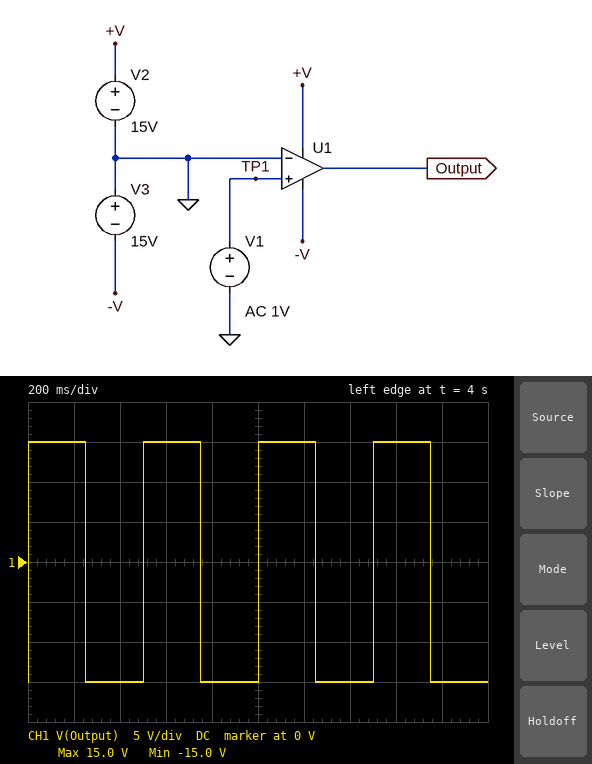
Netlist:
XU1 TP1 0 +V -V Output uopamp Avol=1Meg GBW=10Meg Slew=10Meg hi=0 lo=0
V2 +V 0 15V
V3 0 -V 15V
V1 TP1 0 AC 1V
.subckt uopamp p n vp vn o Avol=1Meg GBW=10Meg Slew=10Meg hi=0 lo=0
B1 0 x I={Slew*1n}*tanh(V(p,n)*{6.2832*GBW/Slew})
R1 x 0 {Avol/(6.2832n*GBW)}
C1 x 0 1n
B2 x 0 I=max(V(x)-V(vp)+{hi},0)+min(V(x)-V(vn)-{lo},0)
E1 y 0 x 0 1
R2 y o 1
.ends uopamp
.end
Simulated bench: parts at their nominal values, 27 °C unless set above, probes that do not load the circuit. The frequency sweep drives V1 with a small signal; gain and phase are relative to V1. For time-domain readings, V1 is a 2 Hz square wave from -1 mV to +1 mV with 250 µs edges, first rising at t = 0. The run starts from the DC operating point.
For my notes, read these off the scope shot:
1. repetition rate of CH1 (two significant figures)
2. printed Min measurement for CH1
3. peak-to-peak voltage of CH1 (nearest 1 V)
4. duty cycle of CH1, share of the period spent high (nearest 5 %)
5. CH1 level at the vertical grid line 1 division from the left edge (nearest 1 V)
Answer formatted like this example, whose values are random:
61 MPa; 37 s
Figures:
2.0 Hz; -15.0 V; 30 V; 50 %; 15 V
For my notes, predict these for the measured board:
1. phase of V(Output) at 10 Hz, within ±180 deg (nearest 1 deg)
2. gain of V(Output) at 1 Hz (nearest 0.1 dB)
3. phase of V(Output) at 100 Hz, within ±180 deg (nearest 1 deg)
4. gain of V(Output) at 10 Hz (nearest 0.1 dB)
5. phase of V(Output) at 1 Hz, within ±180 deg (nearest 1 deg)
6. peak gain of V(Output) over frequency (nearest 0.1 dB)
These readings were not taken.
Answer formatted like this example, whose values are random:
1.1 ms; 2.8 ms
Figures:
-45 deg; 120.0 dB; -84 deg; 117.0 dB; -6 deg; 120.0 dB
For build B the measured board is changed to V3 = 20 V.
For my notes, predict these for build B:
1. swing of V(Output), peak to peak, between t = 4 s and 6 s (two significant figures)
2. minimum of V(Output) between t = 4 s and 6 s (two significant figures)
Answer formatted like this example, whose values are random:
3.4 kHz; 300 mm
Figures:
35 V; -20 V
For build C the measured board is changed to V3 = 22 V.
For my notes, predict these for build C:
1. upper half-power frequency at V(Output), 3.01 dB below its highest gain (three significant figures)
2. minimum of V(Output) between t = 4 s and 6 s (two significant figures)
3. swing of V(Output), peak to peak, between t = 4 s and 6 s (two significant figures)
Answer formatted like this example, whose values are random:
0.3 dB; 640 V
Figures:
10.0 Hz; -22 V; 37 V
